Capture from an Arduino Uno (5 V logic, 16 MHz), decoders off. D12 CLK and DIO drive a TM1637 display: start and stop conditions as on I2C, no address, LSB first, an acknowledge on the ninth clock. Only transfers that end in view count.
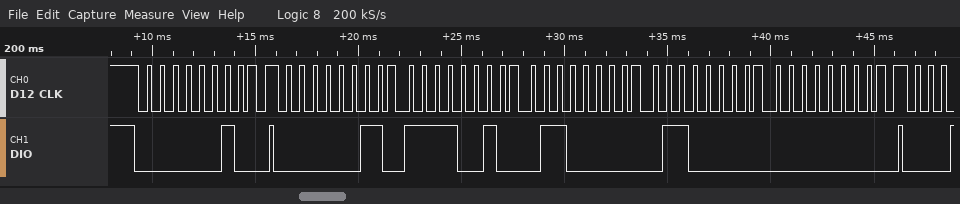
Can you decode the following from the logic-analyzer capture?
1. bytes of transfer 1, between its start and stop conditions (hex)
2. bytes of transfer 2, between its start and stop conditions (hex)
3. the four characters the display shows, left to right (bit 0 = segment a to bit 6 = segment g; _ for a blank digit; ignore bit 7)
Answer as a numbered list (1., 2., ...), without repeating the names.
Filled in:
1. 40
2. C0 4F 06 06 00
3. 311_
